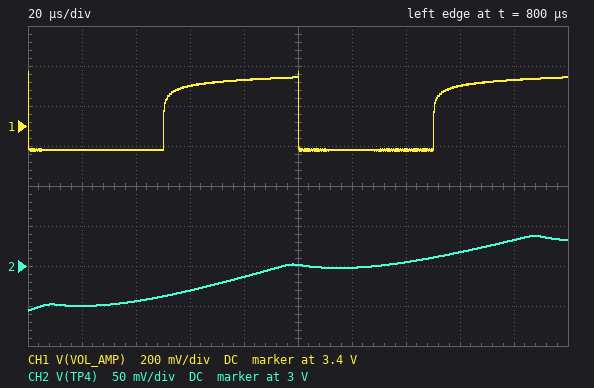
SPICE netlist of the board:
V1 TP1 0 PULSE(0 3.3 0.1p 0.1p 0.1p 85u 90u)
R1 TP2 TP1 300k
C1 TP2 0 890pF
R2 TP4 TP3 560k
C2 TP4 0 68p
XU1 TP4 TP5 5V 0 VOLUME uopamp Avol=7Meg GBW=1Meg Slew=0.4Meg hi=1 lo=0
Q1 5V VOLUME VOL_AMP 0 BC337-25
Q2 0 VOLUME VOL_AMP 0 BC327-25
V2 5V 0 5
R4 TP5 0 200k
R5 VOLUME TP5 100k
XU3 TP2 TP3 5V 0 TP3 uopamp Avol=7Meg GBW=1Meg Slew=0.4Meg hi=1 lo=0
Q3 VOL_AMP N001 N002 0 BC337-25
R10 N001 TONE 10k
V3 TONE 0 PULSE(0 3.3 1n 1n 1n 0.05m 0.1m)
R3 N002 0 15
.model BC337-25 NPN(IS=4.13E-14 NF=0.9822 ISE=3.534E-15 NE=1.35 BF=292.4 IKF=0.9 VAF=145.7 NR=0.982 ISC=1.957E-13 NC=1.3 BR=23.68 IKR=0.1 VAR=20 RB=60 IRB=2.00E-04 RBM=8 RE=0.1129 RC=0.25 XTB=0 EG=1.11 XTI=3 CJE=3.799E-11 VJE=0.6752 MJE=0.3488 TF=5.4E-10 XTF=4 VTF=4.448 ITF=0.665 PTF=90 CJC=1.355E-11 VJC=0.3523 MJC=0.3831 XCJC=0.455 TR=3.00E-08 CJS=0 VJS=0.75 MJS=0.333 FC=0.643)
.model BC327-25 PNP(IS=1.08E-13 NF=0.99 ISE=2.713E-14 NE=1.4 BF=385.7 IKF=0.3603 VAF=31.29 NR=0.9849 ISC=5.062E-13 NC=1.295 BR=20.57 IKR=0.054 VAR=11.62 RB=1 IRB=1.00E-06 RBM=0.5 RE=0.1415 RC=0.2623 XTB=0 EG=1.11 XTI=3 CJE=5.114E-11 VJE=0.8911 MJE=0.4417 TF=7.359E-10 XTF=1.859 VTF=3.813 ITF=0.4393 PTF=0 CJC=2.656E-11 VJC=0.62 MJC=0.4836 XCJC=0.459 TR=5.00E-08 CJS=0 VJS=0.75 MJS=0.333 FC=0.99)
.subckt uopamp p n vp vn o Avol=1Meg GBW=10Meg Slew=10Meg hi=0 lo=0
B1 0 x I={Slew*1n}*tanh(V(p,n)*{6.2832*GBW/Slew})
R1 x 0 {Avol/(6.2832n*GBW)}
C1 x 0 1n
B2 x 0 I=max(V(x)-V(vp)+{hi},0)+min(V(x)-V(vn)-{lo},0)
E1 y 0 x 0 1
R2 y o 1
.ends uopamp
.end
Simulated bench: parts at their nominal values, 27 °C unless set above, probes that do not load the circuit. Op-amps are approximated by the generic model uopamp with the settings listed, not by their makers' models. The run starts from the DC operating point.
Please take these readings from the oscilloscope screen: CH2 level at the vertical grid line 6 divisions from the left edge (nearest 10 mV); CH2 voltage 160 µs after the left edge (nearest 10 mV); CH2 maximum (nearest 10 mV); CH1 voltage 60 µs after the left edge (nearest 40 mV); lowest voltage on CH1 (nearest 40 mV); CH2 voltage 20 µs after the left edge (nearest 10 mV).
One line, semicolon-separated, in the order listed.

3.00 V; 3.02 V; 3.04 V; 3.60 V; 3.28 V; 2.95 V
